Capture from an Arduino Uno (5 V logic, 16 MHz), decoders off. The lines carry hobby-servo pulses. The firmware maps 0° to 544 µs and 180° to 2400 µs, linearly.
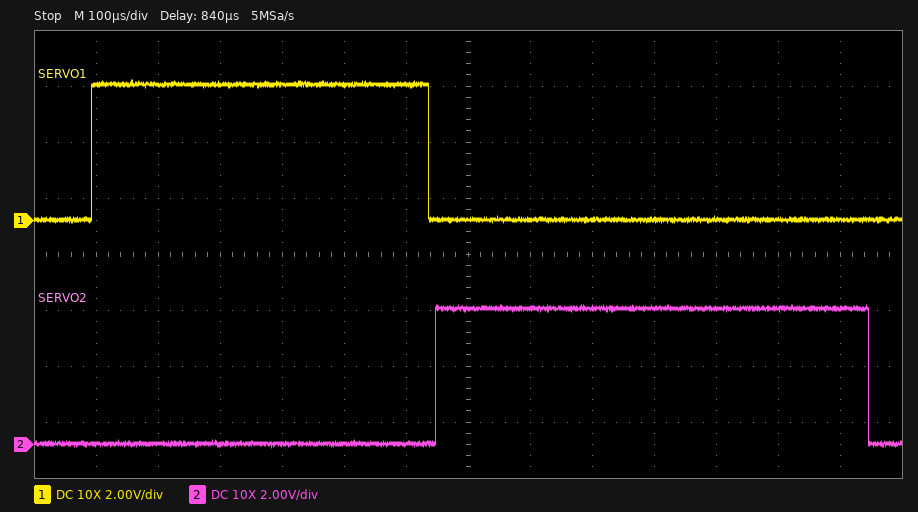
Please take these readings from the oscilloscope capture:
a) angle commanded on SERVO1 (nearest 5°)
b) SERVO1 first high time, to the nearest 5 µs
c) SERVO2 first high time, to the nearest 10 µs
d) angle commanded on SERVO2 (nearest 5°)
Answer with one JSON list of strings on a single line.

["0°", "545 µs", "700 µs", "15°"]
